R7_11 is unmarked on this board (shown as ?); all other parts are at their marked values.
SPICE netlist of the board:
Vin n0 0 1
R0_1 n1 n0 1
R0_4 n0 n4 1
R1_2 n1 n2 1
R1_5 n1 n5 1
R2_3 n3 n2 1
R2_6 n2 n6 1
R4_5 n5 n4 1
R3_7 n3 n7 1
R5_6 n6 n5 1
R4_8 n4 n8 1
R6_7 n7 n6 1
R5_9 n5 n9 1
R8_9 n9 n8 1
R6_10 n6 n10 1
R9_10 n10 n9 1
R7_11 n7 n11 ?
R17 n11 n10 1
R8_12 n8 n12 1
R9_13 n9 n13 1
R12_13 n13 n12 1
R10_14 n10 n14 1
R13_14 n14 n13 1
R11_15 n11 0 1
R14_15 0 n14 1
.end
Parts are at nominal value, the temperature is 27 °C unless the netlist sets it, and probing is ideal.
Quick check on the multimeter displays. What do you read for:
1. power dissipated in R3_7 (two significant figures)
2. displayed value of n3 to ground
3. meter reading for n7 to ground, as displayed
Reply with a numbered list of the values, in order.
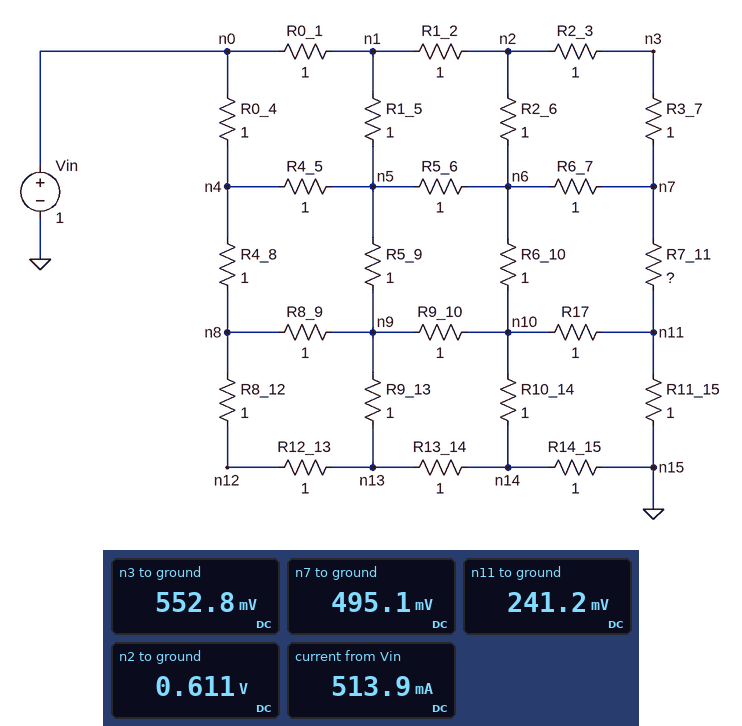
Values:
1. 3.3 mW
2. 552.8 mV
3. 495.1 mV
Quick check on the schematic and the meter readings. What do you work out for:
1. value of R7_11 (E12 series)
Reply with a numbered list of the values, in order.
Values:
1. 2.7 Ω
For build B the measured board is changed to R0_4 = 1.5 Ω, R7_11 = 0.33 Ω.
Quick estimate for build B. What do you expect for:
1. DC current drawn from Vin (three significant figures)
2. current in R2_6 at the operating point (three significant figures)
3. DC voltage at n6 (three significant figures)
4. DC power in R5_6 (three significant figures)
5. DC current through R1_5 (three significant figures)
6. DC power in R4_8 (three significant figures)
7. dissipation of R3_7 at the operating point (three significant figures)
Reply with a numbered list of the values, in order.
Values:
1. 528 mA
2. 78.3 mA
3. 450 mV
4. 13.8 mW
5. 131 mA
6. 17.9 mW
7. 8.47 mW
